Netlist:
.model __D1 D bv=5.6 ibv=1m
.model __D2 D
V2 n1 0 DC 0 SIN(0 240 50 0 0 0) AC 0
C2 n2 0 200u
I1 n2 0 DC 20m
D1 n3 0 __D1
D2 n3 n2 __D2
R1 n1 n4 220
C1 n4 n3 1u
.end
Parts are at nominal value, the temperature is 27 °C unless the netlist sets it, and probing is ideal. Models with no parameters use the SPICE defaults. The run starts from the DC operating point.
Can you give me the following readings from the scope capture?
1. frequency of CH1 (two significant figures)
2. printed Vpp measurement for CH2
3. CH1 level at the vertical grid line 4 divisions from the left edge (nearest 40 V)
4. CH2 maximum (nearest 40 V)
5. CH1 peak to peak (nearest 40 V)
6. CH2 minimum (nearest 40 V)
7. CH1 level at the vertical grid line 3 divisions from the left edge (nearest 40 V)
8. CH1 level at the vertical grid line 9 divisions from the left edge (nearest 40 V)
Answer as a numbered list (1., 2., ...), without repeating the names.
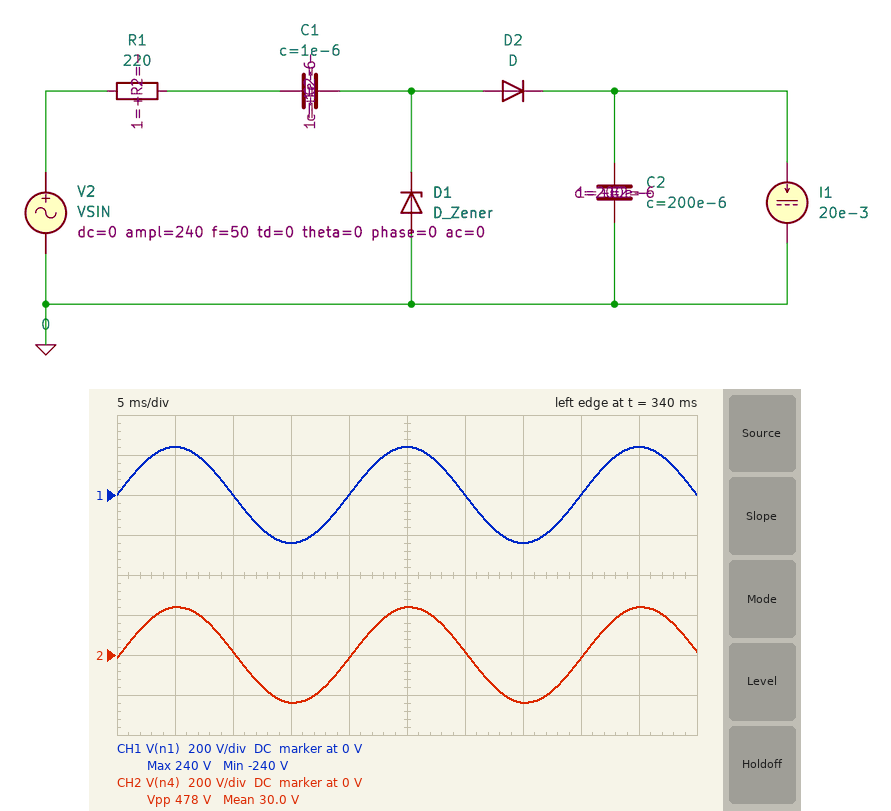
1. 50 Hz
2. 478 V
3. 0 V
4. 240 V
5. 480 V
6. -240 V
7. -240 V
8. 240 V
